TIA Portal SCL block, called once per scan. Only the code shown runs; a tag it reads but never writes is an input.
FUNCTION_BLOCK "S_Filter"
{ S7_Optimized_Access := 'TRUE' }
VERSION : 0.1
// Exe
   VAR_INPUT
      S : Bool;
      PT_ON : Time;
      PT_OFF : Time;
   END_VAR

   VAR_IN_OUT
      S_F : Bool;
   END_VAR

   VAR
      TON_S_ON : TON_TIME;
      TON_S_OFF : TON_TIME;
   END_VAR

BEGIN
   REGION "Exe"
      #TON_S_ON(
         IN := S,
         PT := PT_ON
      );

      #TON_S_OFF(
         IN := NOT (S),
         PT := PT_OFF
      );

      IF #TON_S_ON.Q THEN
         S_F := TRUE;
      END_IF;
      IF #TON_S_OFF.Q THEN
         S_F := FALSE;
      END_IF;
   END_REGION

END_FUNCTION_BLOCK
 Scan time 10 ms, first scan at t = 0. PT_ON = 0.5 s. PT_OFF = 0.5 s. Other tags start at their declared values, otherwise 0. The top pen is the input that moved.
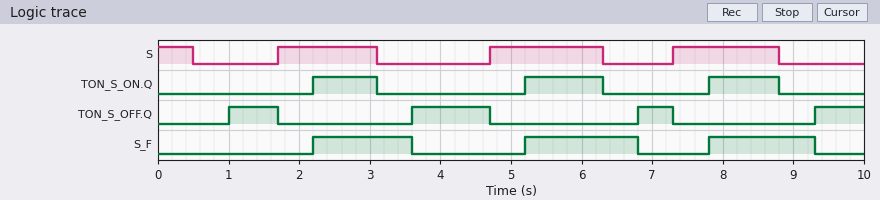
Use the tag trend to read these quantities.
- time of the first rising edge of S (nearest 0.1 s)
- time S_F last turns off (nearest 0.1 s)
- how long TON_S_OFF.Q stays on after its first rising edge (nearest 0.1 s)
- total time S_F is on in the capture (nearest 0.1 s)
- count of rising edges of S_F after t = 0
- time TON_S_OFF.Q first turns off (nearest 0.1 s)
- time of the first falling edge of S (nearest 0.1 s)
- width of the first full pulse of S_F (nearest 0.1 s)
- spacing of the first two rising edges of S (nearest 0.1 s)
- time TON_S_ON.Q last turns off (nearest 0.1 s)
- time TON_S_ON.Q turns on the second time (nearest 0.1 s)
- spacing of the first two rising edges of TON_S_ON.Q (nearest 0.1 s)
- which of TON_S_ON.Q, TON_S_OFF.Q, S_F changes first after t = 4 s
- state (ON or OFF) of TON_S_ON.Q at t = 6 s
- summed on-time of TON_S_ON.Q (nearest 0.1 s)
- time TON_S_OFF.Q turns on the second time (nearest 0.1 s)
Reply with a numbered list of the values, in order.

1. 1.7 s
2. 9.3 s
3. 0.7 s
4. 4.5 s
5. 3
6. 1.7 s
7. 0.5 s
8. 1.4 s
9. 3.0 s
10. 8.8 s
11. 5.2 s
12. 3.0 s
13. TON_S_OFF.Q
14. ON
15. 3.0 s
16. 3.6 s
